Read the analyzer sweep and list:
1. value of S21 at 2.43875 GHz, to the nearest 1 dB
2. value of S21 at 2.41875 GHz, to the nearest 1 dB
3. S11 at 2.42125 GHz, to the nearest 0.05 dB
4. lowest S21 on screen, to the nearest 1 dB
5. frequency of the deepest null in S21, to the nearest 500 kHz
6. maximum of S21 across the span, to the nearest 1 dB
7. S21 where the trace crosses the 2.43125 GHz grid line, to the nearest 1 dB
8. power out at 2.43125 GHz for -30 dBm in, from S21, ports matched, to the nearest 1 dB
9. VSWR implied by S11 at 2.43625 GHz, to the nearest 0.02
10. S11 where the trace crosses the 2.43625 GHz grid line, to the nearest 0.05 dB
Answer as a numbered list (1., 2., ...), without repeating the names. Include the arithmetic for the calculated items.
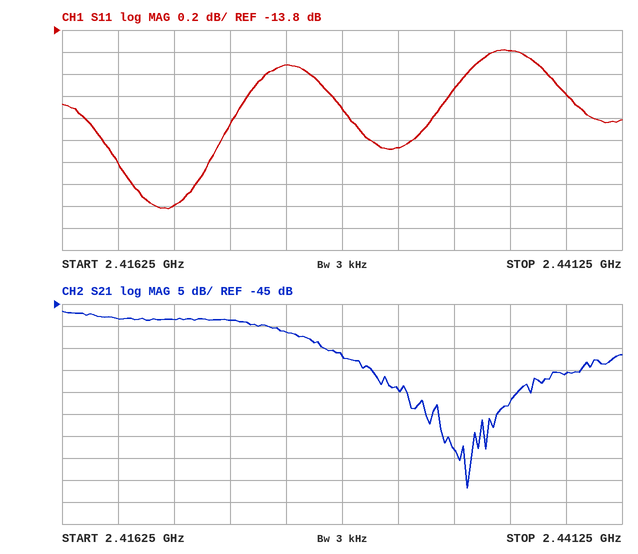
1. -61 dB
2. -48 dB
3. -15.40 dB
4. -87 dB
5. 2.4345 GHz
6. -47 dB
7. -64 dB
8. -30 dBm + (-64 dB) = -94 dBm
9. |Γ| = 10^(-14/20) = 0.1995; VSWR = (1 + 0.1995)/(1 − 0.1995) ≈ 1.50
10. -14.00 dB
